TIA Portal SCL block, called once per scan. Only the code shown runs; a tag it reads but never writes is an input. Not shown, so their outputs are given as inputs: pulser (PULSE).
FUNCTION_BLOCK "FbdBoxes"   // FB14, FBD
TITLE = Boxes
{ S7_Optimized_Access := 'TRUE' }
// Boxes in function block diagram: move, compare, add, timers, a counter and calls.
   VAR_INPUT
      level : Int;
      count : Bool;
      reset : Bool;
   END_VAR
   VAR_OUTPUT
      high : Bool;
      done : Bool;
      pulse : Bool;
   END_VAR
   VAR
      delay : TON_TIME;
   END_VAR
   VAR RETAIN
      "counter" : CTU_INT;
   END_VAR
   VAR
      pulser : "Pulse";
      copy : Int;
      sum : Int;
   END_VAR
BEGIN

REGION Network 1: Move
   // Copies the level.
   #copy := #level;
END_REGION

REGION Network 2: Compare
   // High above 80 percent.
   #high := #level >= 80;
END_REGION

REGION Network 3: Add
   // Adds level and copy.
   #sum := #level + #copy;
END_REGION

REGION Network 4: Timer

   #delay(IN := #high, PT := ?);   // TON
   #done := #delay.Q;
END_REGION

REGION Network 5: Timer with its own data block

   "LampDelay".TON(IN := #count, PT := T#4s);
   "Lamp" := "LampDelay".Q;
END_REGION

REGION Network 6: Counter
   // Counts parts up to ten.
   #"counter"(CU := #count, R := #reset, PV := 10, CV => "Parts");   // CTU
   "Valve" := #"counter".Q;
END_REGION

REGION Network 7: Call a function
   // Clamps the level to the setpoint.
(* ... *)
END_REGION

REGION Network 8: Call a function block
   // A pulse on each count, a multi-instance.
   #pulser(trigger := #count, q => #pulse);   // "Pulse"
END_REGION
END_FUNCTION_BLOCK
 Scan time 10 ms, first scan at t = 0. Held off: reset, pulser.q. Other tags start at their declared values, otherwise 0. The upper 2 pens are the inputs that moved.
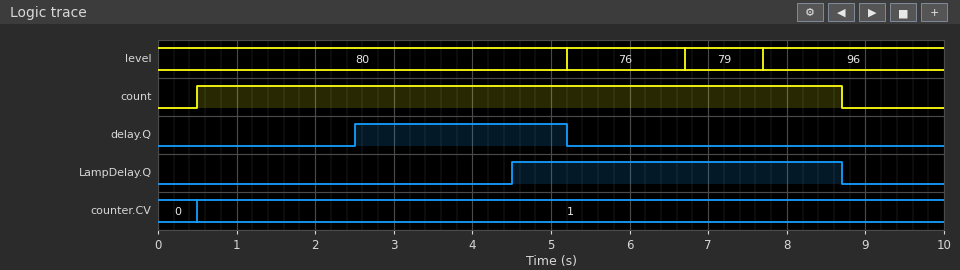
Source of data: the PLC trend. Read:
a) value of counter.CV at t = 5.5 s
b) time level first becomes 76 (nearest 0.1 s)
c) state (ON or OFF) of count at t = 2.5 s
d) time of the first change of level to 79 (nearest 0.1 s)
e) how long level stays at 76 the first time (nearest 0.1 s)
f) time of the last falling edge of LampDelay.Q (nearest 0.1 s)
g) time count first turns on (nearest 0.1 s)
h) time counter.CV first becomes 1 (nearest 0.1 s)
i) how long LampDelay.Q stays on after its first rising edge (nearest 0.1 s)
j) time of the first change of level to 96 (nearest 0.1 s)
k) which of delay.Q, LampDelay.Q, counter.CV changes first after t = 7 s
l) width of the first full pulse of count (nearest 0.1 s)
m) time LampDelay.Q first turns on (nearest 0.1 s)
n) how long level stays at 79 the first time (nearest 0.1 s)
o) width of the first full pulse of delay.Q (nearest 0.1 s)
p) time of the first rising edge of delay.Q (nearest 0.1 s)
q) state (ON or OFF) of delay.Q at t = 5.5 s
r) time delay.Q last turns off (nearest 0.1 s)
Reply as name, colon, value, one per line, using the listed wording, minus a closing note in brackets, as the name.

value of counter.CV at t = 5.5 s: 1
time level first becomes 76: 5.2 s
state (ON or OFF) of count at t = 2.5 s: ON
time of the first change of level to 79: 6.7 s
how long level stays at 76 the first time: 1.5 s
time of the last falling edge of LampDelay.Q: 8.7 s
time count first turns on: 0.5 s
time counter.CV first becomes 1: 0.5 s
how long LampDelay.Q stays on after its first rising edge: 4.2 s
time of the first change of level to 96: 7.7 s
which of delay.Q, LampDelay.Q, counter.CV changes first after t = 7 s: LampDelay.Q
width of the first full pulse of count: 8.2 s
time LampDelay.Q first turns on: 4.5 s
how long level stays at 79 the first time: 1.0 s
width of the first full pulse of delay.Q: 2.7 s
time of the first rising edge of delay.Q: 2.5 s
state (ON or OFF) of delay.Q at t = 5.5 s: OFF
time delay.Q last turns off: 5.2 s
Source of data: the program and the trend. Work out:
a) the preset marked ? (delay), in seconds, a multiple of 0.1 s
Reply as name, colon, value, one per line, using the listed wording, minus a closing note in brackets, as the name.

the preset marked ? (delay), in seconds, a multiple of 0.1 s: 2.5 s
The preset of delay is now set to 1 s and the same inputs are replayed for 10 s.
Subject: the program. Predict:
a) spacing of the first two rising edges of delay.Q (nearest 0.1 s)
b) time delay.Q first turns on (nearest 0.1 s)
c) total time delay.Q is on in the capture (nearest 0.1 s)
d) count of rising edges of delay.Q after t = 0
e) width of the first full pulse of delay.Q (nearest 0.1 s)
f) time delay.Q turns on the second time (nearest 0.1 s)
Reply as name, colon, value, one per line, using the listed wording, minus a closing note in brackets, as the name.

spacing of the first two rising edges of delay.Q: 7.7 s
time delay.Q first turns on: 1.0 s
total time delay.Q is on in the capture: 5.5 s
count of rising edges of delay.Q after t = 0: 2
width of the first full pulse of delay.Q: 4.2 s
time delay.Q turns on the second time: 8.7 s
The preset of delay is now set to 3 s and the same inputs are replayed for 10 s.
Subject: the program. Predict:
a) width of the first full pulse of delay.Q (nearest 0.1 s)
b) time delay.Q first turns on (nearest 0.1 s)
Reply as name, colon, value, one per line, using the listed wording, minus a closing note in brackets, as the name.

width of the first full pulse of delay.Q: 2.2 s
time delay.Q first turns on: 3.0 s
